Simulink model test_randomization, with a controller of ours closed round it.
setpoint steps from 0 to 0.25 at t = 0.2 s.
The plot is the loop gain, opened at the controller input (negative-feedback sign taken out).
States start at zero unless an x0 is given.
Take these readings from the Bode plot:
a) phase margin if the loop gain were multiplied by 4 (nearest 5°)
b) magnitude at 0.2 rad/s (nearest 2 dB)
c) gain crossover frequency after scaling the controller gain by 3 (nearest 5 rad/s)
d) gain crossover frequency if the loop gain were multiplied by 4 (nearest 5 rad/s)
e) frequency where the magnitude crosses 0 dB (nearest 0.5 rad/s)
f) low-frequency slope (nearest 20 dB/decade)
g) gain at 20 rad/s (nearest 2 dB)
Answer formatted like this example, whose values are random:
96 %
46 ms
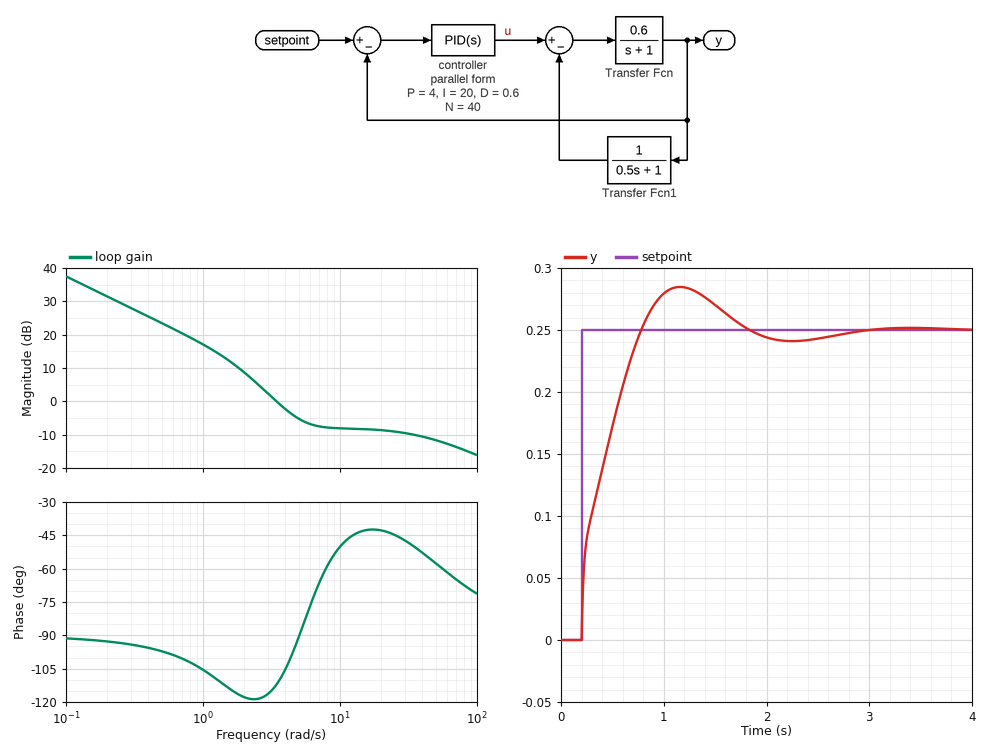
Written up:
120°
32 dB
30 rad/s
55 rad/s
3.5 rad/s
-20 dB/decade
-8 dB
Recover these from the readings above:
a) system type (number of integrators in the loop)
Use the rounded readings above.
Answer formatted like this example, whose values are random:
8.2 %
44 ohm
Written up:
1
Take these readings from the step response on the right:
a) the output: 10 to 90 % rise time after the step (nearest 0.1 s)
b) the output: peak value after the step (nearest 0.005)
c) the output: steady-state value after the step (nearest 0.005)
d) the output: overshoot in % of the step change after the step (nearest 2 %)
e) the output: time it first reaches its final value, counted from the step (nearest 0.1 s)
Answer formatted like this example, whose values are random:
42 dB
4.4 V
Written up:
0.5 s
0.285
0.250
14 %
0.6 s
